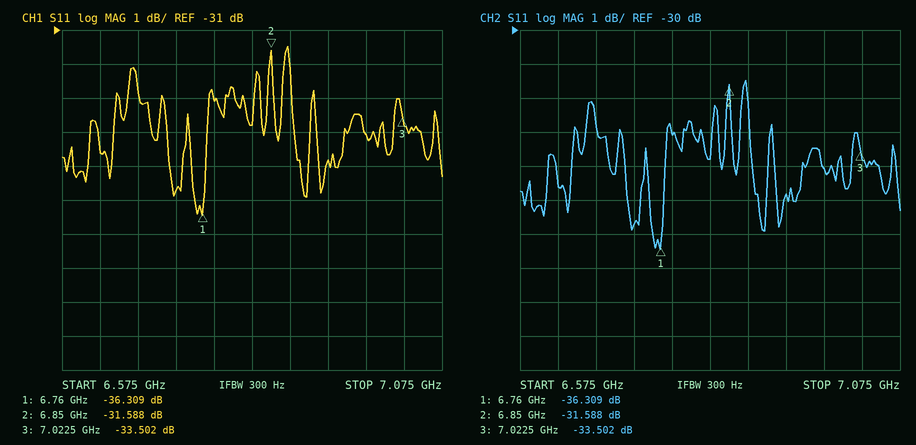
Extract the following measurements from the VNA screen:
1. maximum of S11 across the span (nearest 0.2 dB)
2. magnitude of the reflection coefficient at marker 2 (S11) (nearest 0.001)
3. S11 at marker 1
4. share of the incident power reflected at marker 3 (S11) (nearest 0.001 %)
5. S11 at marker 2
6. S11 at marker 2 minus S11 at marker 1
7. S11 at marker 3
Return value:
-31.4 dB
0.026
-36.309 dB
0.045 %
-31.588 dB
4.721 dB
-33.502 dB
